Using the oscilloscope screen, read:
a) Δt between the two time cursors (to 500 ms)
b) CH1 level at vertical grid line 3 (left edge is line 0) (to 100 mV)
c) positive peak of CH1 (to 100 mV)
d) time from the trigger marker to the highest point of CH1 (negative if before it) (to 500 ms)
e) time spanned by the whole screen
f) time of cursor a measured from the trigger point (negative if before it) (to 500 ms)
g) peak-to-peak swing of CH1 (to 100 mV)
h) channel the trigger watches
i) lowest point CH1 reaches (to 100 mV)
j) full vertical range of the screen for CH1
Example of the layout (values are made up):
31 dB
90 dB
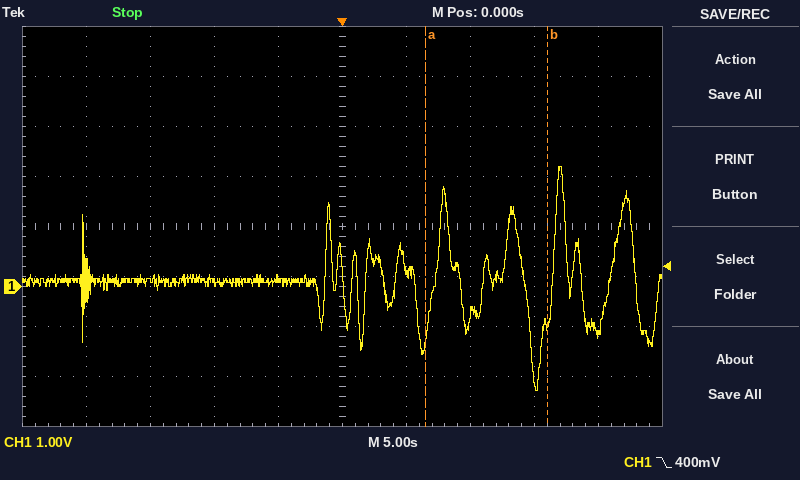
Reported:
9.5 s
100 mV
2.4 V
+17.0 s
50 s
+6.5 s
4.5 V
CH1
-2.1 V
8 V
